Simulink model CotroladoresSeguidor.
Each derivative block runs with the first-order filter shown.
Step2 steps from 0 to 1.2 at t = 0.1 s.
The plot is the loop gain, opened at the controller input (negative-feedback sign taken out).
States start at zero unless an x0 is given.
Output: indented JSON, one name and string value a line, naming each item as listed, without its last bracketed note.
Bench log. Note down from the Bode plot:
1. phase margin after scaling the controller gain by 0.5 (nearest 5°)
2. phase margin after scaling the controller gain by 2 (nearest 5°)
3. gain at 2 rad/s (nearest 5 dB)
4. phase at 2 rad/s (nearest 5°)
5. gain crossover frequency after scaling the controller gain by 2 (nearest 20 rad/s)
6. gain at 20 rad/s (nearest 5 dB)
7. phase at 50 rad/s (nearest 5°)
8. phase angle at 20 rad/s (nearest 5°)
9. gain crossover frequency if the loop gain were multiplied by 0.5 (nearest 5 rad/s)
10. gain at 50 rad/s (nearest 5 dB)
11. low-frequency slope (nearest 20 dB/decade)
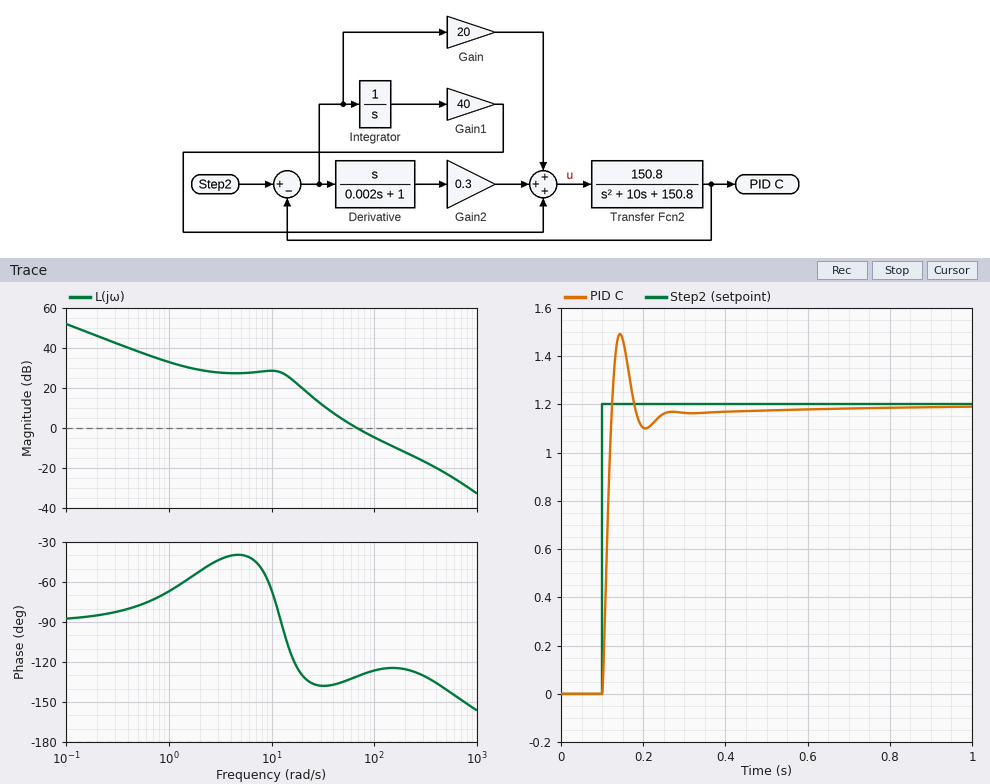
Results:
{
  "phase margin after scaling the controller gain by 0.5": "45°",
  "phase margin after scaling the controller gain by 2": "55°",
  "gain at 2 rad/s": "30 dB",
  "phase at 2 rad/s": "-50°",
  "gain crossover frequency after scaling the controller gain by 2": "120 rad/s",
  "gain at 20 rad/s": "20 dB",
  "phase at 50 rad/s": "-135°",
  "phase angle at 20 rad/s": "-130°",
  "gain crossover frequency if the loop gain were multiplied by 0.5": "45 rad/s",
  "gain at 50 rad/s": "5 dB",
  "low-frequency slope": "-20 dB/decade"
}
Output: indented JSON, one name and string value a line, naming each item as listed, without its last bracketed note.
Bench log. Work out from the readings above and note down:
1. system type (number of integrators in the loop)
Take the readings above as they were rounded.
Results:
{
  "system type": "1"
}
